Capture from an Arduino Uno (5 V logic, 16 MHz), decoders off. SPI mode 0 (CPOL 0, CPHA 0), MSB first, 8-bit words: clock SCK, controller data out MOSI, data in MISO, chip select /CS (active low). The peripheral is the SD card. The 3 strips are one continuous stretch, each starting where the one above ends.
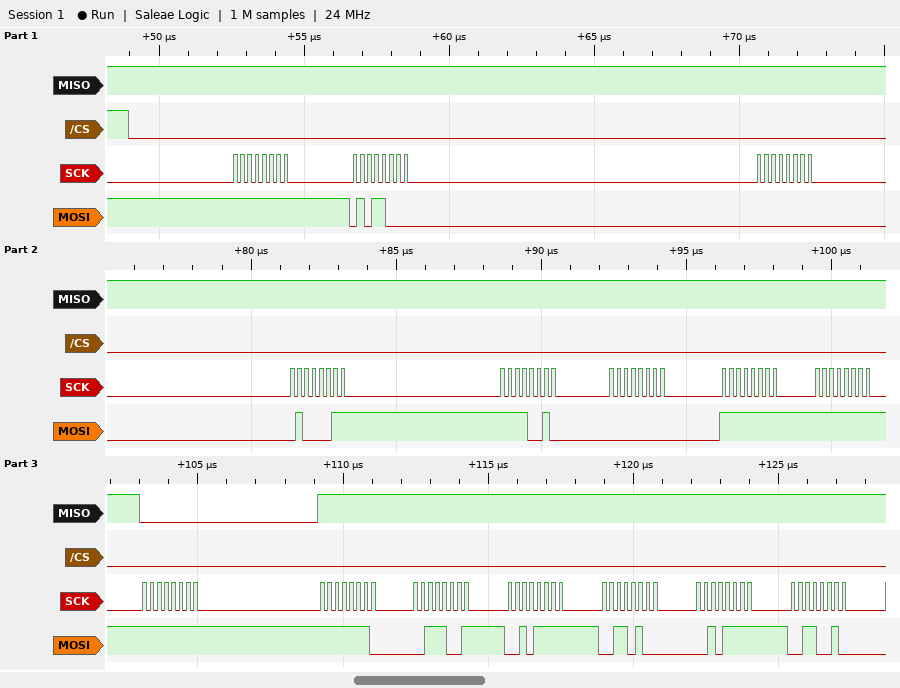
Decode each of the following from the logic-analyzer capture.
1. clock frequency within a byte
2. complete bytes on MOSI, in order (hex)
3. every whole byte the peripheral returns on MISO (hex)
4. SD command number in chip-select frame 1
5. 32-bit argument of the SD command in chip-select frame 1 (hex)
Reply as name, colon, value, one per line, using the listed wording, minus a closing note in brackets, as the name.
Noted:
clock frequency within a byte: 4 MHz
complete bytes on MOSI, in order: FF 58 00 43 F2 00 FF FF FF FE 39 2F 34 2F 32
every whole byte the peripheral returns on MISO: FF FF FF FF FF FF FF FF 00 FF FF FF FF FF FF
SD command number in chip-select frame 1: CMD24
32-bit argument of the SD command in chip-select frame 1: 0x0043F200
